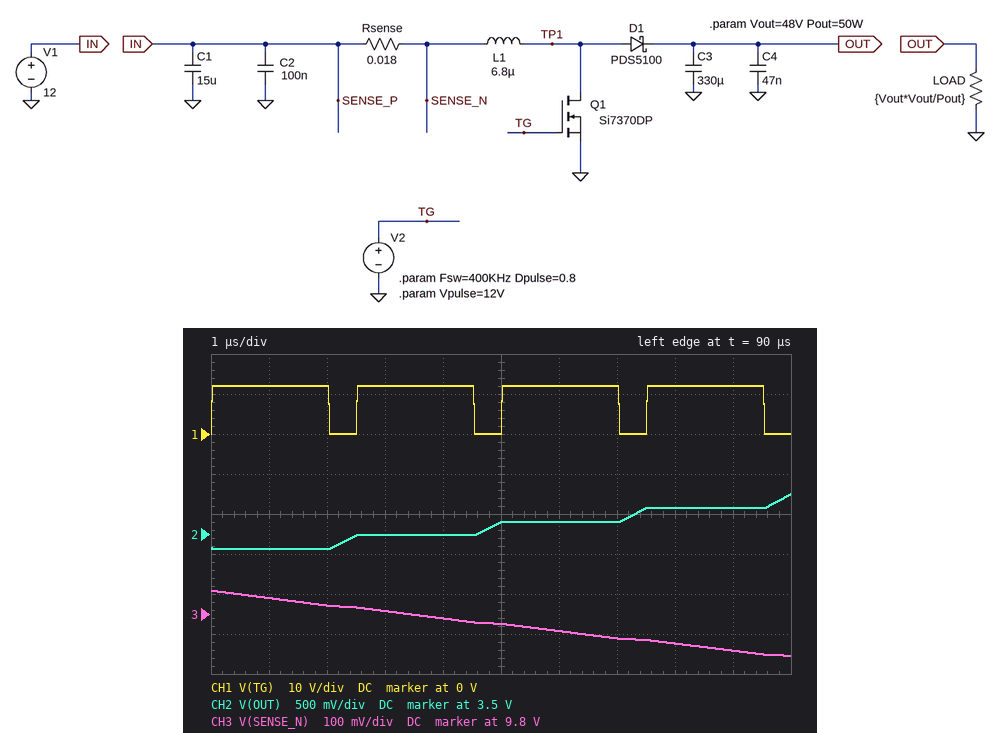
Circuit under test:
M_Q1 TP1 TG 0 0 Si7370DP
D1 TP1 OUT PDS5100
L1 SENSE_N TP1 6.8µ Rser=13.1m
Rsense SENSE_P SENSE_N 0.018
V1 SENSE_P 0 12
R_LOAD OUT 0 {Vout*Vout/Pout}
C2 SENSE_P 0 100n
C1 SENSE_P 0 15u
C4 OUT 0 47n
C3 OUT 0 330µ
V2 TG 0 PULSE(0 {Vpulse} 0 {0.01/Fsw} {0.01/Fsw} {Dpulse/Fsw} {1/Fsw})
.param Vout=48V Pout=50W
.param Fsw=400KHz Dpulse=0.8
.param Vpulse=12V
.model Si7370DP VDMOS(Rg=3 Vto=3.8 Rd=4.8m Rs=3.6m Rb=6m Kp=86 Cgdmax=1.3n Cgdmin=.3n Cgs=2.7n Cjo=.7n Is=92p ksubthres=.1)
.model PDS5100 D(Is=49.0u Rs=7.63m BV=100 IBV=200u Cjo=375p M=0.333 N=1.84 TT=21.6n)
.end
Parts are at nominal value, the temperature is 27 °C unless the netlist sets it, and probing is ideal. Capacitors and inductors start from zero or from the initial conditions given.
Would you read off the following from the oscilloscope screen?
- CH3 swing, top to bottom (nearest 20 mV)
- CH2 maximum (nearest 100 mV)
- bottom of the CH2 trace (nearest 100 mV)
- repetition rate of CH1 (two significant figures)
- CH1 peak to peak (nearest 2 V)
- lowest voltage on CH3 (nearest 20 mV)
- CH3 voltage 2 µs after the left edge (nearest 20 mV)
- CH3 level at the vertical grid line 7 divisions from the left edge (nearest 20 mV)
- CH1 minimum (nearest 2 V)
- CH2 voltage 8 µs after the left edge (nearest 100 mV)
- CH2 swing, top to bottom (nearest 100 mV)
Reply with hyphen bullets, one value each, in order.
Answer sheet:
- 160 mV
- 4.0 V
- 3.3 V
- 400 kHz
- 12 V
- 9.70 V
- 9.82 V
- 9.74 V
- 0 V
- 3.8 V
- 700 mV
